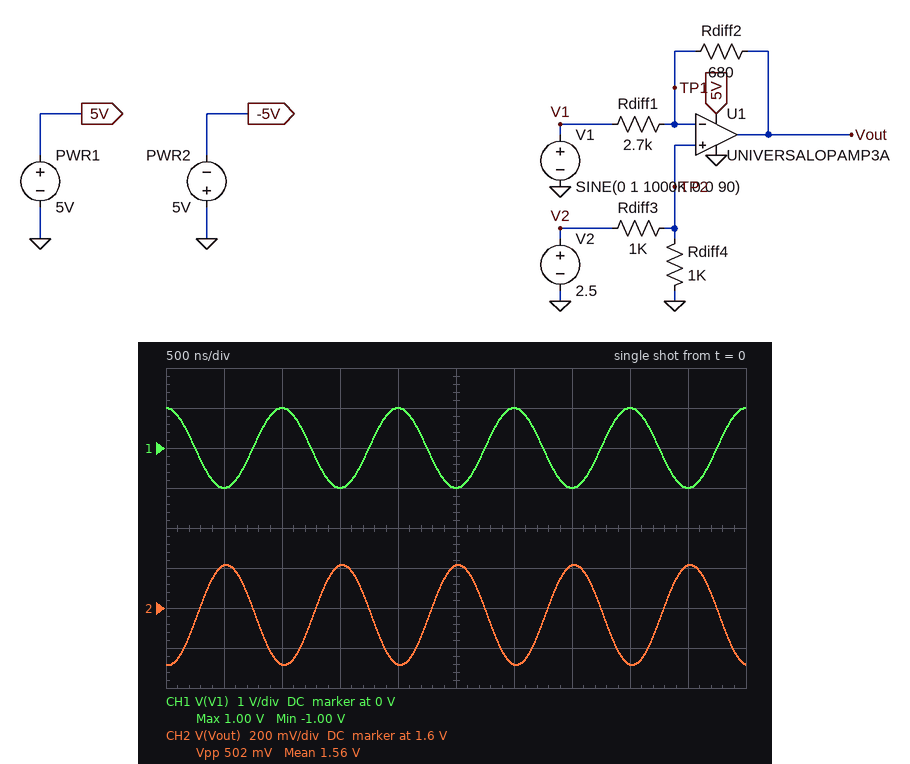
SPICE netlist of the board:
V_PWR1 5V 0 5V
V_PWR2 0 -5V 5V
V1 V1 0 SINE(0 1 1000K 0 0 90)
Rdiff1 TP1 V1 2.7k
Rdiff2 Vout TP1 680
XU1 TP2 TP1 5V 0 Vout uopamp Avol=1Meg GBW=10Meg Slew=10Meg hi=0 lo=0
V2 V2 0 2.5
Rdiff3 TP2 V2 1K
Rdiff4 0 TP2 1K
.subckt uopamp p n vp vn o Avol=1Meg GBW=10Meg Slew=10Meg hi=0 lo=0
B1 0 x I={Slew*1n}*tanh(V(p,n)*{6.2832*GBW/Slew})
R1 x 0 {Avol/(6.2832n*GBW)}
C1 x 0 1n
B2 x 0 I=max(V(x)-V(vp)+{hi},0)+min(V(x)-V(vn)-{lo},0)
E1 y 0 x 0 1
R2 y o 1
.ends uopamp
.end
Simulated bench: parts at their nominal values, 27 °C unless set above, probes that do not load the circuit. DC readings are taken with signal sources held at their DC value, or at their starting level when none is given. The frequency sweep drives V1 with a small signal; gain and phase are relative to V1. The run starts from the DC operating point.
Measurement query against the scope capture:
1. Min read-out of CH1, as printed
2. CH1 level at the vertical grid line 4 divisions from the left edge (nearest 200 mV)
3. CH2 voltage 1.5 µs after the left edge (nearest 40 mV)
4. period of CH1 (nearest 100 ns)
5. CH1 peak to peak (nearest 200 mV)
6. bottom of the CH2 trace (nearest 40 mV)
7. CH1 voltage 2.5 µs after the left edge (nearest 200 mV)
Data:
-1.00 V
1.0 V
1.80 V
1.0 µs
2.0 V
1.32 V
-1.0 V
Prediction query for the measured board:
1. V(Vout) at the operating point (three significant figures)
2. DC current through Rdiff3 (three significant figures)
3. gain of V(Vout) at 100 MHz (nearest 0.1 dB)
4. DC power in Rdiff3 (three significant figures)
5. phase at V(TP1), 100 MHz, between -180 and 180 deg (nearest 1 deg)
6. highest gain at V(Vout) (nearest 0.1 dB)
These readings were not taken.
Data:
1.31 V
1.25 mA
-34.0 dB
1.56 mW
5 deg
-12.0 dB
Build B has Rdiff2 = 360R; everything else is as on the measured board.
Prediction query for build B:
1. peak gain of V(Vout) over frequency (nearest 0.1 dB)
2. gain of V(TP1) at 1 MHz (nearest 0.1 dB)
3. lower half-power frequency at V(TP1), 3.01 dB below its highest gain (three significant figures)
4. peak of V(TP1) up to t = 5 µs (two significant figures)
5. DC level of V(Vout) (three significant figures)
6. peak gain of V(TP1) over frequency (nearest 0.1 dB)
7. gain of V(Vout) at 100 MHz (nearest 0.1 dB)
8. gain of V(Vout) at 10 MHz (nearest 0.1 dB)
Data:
-17.5 dB
-37.5 dB
8.82 MHz
1.3 V
1.28 V
-18.6 dB
-38.6 dB
-21.1 dB
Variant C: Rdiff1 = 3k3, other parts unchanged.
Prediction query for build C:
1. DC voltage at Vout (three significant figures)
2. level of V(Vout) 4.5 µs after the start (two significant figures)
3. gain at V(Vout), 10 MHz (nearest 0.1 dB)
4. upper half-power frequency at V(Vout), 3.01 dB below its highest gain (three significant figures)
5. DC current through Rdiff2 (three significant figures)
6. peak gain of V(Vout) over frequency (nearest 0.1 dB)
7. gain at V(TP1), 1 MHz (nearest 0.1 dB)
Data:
1.30 V
1.7 V
-17.6 dB
8.29 MHz
75.8 µA
-13.7 dB
-33.8 dB
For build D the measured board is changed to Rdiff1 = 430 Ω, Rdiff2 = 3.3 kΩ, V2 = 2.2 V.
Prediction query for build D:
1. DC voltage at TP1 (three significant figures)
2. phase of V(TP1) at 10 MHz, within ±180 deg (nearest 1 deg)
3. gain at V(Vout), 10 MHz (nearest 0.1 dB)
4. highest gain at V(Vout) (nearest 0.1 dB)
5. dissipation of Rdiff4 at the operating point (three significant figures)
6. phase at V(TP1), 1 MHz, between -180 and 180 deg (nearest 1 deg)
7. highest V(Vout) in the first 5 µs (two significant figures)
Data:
1.10 V
7 deg
-1.1 dB
17.7 dB
1.21 mW
49 deg
5.0 V
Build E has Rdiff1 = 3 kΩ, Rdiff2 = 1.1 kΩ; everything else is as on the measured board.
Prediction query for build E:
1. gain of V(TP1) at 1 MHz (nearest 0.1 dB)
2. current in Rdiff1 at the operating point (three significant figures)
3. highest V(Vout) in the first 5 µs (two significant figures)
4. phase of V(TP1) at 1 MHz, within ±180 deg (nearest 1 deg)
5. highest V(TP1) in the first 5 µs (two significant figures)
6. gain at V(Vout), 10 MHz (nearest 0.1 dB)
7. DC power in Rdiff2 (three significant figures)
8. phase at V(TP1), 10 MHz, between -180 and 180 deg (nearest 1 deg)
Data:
-28.8 dB
83.3 µA
2.1 V
82 deg
1.3 V
-13.3 dB
7.64 µW
36 deg
